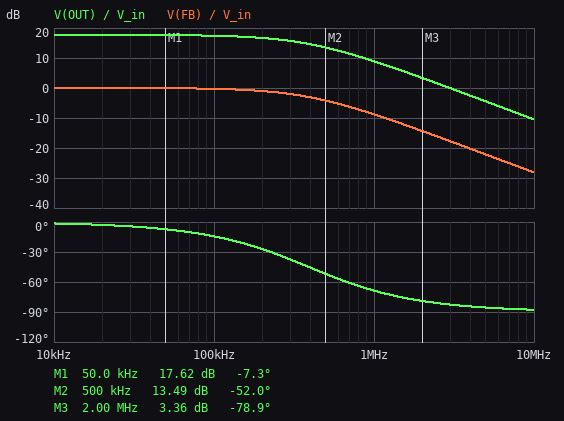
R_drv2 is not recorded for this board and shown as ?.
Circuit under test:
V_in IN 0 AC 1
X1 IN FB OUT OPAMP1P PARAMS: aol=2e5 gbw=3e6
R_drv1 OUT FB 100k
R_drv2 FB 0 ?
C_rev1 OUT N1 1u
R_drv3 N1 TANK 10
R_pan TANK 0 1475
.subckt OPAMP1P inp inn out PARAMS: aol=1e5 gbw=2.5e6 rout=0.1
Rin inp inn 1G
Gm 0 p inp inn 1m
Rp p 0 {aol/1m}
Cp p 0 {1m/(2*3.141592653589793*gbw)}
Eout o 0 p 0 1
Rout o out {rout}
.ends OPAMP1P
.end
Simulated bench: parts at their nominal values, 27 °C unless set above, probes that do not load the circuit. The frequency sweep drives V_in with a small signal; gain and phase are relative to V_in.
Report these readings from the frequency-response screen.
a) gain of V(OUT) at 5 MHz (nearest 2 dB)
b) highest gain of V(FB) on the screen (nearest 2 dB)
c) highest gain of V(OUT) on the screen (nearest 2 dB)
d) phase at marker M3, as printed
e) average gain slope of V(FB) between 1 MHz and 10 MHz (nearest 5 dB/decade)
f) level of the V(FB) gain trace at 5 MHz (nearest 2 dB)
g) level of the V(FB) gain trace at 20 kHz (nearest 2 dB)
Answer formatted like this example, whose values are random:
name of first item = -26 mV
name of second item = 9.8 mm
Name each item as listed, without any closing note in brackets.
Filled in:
gain of V(OUT) at 5 MHz = -4 dB
highest gain of V(FB) on the screen = 0 dB
highest gain of V(OUT) on the screen = 18 dB
phase at marker M3, as printed = -78.9 deg
average gain slope of V(FB) between 1 MHz and 10 MHz = -20 dB/decade
level of the V(FB) gain trace at 5 MHz = -22 dB
level of the V(FB) gain trace at 20 kHz = 0 dB
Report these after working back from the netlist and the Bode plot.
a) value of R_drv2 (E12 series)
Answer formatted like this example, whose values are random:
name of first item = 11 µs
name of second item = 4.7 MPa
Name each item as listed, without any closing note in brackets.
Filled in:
value of R_drv2 = 15 kΩ
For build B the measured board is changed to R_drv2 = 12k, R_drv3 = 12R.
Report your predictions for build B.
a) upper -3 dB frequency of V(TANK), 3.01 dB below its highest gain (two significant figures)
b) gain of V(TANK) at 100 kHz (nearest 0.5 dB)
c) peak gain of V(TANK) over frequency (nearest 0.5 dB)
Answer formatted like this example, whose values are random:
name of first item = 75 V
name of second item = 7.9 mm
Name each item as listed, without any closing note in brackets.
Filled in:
upper -3 dB frequency of V(TANK), 3.01 dB below its highest gain = 320 kHz
gain of V(TANK) at 100 kHz = 19.0 dB
peak gain of V(TANK) over frequency = 19.5 dB
